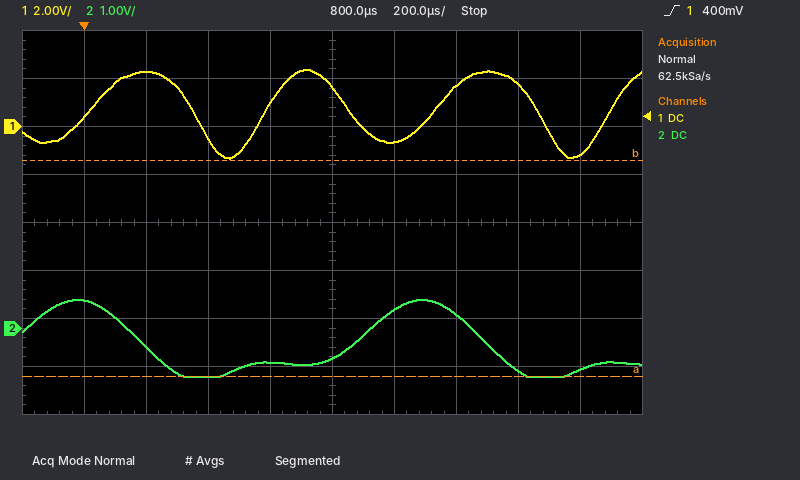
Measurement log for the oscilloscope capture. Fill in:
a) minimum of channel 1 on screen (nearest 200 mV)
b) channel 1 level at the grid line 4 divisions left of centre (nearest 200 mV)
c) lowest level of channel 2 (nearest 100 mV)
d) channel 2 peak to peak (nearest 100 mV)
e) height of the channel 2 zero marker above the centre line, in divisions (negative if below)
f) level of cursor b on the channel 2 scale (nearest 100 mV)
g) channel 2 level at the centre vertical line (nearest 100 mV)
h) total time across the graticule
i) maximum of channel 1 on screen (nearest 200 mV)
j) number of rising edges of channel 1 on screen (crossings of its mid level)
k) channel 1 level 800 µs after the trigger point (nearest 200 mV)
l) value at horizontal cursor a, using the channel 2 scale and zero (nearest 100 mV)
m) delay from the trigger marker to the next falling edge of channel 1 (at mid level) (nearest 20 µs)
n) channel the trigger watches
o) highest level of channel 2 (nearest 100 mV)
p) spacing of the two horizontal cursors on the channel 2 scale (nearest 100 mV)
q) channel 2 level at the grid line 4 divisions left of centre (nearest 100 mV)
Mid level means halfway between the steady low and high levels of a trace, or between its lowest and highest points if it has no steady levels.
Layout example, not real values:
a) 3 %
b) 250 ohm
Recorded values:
a) -1.4 V
b) 400 mV
c) -1.0 V
d) 1.6 V
e) -2.2 div
f) 3.5 V
g) -600 mV
h) 2 ms
i) 2.4 V
j) 4
k) 1.6 V
l) -1.0 V
m) 360 µs
n) channel 1
o) 600 mV
p) 4.5 V
q) 600 mV
